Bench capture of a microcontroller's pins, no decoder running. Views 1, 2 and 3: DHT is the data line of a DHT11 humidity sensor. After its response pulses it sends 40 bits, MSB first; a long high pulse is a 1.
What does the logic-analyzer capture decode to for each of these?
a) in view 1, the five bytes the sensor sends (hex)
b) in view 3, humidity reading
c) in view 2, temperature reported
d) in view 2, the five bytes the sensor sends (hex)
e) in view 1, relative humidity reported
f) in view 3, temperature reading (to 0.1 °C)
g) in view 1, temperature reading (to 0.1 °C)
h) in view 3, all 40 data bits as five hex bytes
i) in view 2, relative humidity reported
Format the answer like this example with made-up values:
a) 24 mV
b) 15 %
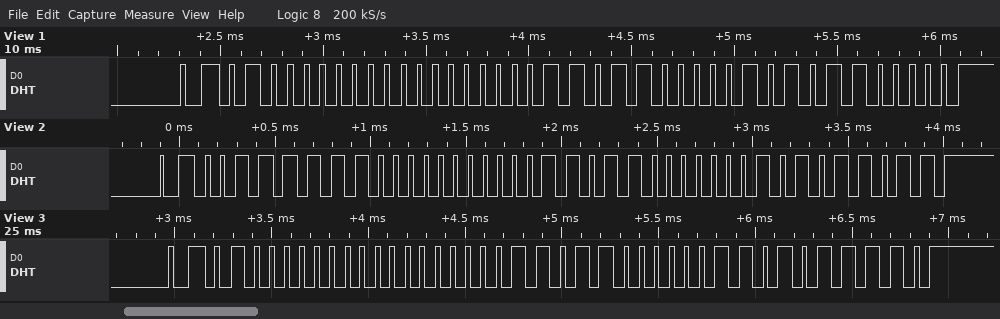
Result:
a) 40 00 1B 05 60
b) 64 %
c) 27.1 °C
d) 3F 00 1B 01 5B
e) 64 %
f) 27.3 °C
g) 27.5 °C
h) 40 00 1B 03 5E
i) 63 %
